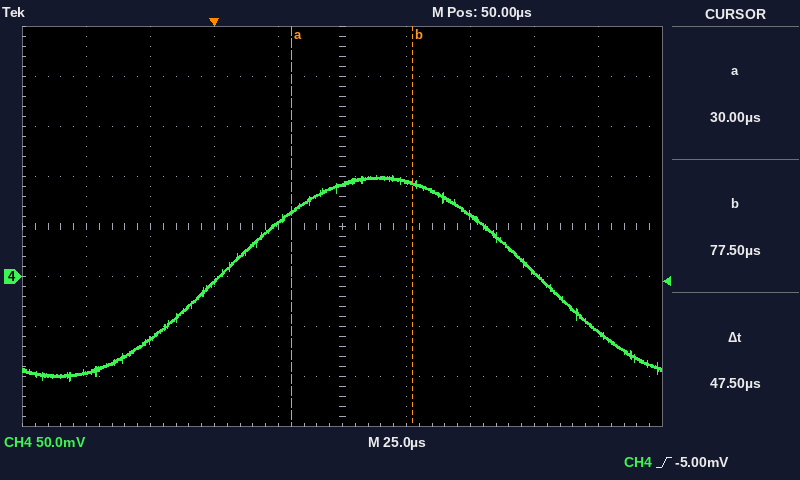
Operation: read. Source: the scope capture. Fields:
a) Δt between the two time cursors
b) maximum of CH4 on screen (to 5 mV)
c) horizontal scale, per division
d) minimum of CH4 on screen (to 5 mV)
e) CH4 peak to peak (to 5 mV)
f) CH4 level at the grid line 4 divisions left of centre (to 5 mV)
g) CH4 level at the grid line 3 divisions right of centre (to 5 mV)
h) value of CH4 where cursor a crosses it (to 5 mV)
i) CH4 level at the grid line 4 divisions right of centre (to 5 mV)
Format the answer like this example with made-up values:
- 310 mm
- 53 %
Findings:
- 47.5 µs
- 100 mV
- 25 µs
- -105 mV
- 205 mV
- -95 mV
- 5 mV
- 65 mV
- -55 mV
